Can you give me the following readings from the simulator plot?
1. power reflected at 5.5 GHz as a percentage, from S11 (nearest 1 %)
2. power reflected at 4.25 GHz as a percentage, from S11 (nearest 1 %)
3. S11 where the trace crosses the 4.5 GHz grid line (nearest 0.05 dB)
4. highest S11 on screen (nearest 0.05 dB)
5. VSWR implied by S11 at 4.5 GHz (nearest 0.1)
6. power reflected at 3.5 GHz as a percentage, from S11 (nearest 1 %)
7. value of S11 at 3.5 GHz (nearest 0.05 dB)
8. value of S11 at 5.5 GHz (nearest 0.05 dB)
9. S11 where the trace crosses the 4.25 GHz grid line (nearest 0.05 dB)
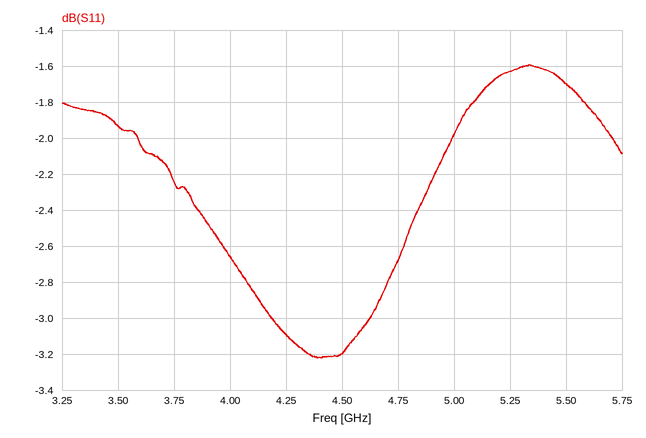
68 %
49 %
-3.20 dB
-1.60 dB
5.5
64 %
-1.95 dB
-1.70 dB
-3.10 dB
